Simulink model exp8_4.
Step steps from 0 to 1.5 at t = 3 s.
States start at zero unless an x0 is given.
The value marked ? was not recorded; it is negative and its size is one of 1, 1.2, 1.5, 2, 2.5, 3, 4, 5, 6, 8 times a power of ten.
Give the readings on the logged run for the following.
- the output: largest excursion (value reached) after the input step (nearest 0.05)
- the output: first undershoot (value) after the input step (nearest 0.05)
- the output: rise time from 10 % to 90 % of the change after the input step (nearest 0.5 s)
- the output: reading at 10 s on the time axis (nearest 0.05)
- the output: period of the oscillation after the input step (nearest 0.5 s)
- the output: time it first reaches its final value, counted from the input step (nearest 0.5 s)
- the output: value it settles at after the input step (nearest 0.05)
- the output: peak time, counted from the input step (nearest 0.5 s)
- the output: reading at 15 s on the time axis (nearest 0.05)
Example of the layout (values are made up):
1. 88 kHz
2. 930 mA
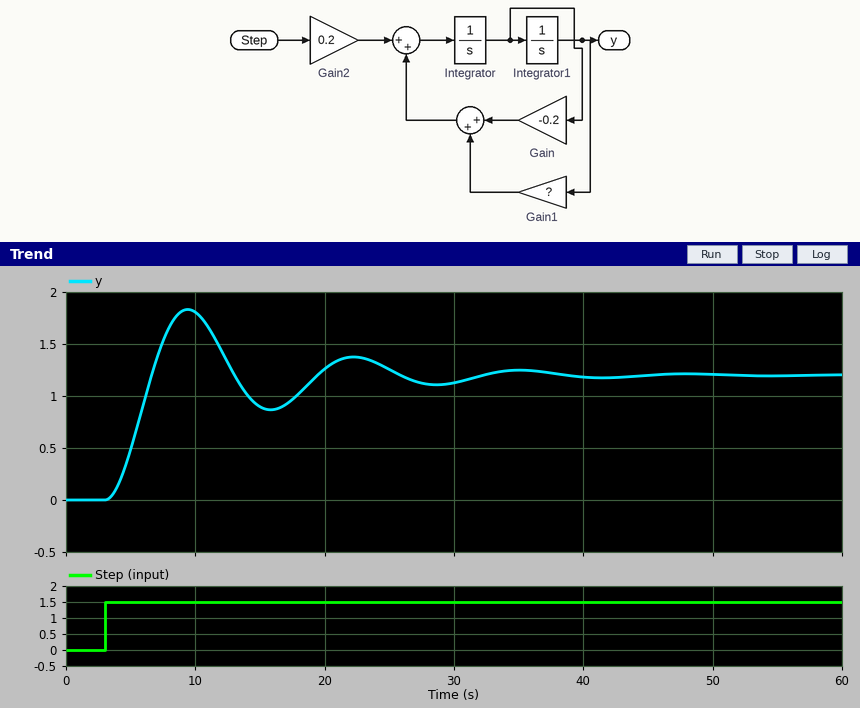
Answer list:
1. 1.85
2. 0.85
3. 2.5 s
4. 1.80
5. 13.0 s
6. 3.5 s
7. 1.20
8. 6.5 s
9. 0.90
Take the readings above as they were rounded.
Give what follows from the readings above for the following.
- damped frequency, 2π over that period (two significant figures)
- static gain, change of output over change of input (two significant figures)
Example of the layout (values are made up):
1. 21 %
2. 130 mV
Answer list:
1. 0.48 rad/s
2. 0.80
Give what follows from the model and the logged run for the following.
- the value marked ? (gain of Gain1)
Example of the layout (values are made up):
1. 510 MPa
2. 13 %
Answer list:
1. -0.25
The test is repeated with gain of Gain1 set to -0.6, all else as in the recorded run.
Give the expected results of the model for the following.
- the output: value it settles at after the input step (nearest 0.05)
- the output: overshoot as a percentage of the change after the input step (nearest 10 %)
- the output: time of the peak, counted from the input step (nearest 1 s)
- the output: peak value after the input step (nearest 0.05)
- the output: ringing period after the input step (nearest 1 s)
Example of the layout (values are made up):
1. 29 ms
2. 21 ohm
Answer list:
1. 0.50
2. 70 %
3. 4 s
4. 0.85
5. 8 s
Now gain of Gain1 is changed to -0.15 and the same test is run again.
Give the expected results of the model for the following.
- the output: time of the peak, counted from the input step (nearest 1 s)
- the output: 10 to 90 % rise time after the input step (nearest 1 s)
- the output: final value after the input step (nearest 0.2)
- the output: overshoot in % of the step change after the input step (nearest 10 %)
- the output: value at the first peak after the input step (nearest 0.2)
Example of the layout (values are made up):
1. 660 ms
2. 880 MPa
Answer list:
1. 8 s
2. 3 s
3. 2.0
4. 40 %
5. 2.8
